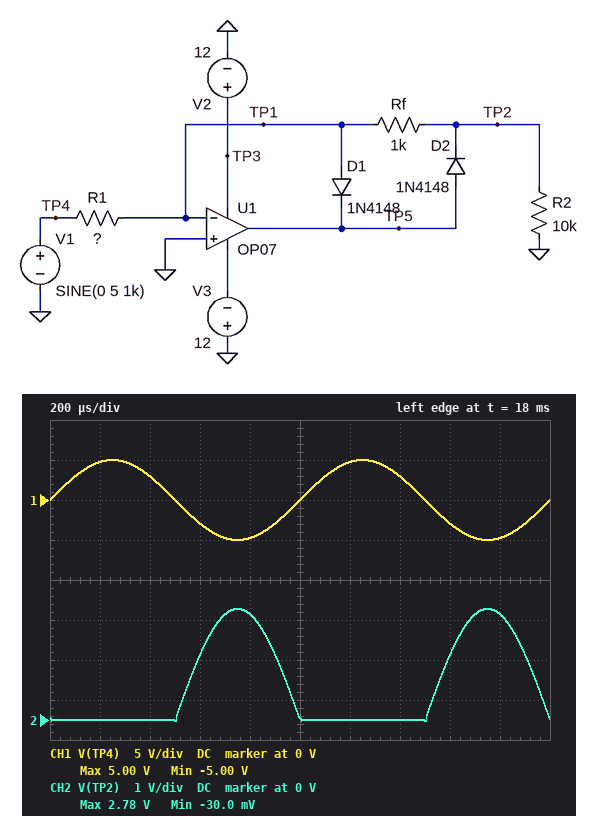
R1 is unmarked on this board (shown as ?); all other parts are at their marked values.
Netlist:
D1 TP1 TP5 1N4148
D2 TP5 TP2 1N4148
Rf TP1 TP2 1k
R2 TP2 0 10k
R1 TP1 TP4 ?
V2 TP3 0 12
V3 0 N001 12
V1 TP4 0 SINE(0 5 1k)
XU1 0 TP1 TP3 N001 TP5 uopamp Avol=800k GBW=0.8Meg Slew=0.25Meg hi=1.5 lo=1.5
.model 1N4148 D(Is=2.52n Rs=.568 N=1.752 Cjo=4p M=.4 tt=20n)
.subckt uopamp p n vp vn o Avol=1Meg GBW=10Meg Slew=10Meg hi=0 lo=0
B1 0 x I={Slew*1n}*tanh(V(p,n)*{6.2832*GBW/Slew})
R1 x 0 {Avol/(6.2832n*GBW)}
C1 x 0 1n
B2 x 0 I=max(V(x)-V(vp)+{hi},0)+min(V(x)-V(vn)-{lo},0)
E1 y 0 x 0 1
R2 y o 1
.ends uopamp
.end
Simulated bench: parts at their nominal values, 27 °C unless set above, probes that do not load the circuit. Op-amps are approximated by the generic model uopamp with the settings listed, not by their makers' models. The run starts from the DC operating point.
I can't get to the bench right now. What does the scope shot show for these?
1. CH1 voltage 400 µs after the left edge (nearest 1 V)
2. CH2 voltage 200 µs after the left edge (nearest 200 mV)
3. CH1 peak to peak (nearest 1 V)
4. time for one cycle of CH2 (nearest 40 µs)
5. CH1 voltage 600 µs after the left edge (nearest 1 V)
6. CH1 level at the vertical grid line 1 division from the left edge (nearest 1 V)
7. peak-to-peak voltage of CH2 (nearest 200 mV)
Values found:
3 V
0 V
10 V
1.00 ms
-3 V
5 V
2.8 V
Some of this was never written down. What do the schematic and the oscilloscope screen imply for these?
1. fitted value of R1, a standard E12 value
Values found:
1.8 kΩ
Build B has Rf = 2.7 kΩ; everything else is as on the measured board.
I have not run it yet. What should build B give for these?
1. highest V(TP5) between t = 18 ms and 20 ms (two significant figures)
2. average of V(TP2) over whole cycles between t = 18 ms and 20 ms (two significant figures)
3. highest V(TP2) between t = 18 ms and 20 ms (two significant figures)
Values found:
8.1 V
2.4 V
7.5 V
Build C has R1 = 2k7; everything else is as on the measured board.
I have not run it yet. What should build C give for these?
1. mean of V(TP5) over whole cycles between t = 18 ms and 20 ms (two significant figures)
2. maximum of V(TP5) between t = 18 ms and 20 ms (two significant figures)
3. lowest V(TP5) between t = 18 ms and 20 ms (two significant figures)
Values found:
590 mV
2.5 V
-610 mV
